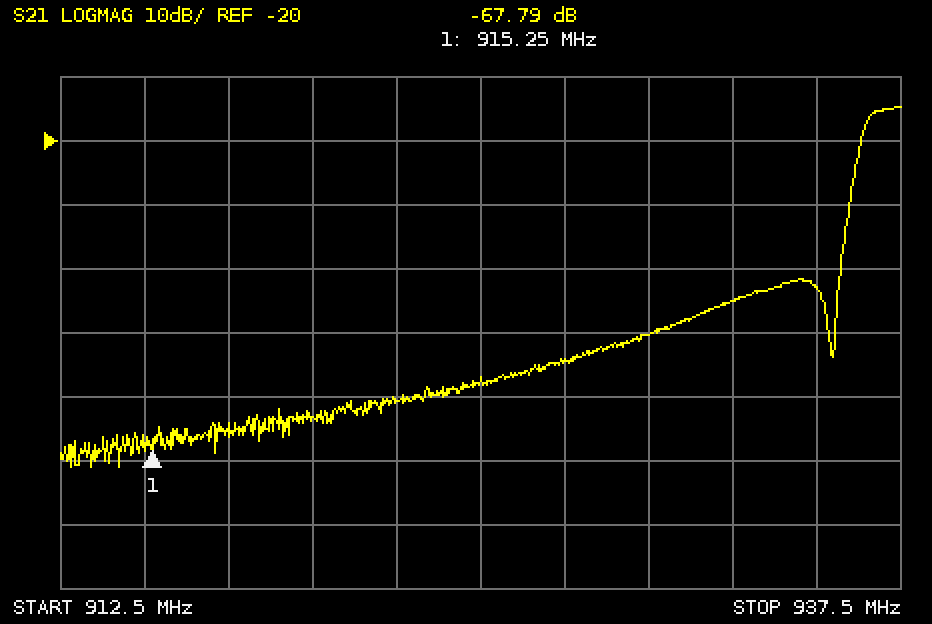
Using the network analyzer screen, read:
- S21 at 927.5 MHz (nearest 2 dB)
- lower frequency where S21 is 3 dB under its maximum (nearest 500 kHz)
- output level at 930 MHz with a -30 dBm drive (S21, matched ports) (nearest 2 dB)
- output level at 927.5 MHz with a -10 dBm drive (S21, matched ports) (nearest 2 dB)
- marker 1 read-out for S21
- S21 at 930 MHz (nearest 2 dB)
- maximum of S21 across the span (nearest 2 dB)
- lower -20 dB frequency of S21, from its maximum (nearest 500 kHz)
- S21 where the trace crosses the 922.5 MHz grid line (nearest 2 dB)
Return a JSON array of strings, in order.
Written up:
["-54 dB", "936.5 MHz", "-80 dBm", "-64 dBm", "-67.79 dB", "-50 dB", "-14 dB", "936.0 MHz", "-60 dB"]
